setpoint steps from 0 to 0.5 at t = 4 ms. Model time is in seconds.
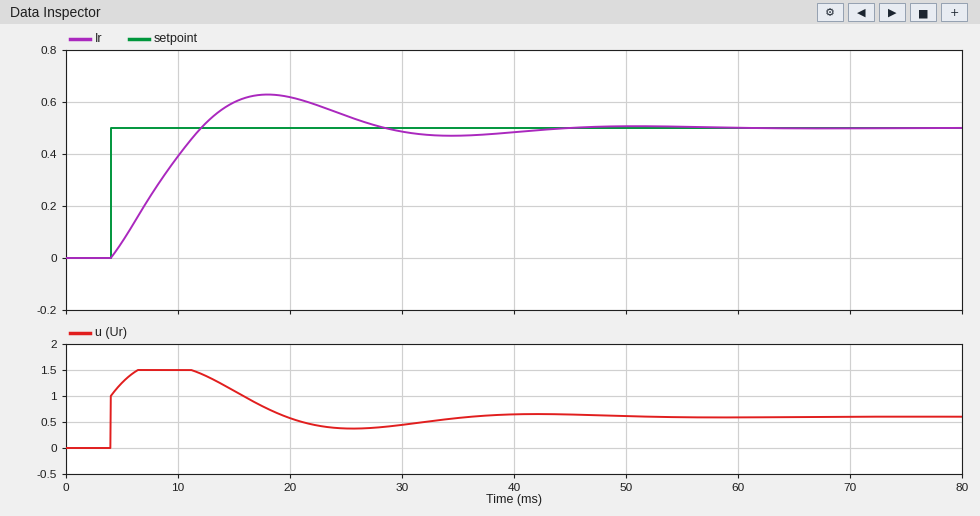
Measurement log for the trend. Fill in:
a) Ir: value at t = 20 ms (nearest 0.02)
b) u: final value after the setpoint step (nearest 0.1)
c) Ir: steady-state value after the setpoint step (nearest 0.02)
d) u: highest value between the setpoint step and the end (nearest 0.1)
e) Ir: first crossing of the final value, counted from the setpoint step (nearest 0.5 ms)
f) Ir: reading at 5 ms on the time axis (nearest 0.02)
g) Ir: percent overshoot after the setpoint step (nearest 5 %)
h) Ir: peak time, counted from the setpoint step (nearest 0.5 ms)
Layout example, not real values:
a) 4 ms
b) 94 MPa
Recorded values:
a) 0.62
b) 0.6
c) 0.50
d) 1.5
e) 8.0 ms
f) 0.06
g) 25 %
h) 14.0 ms
